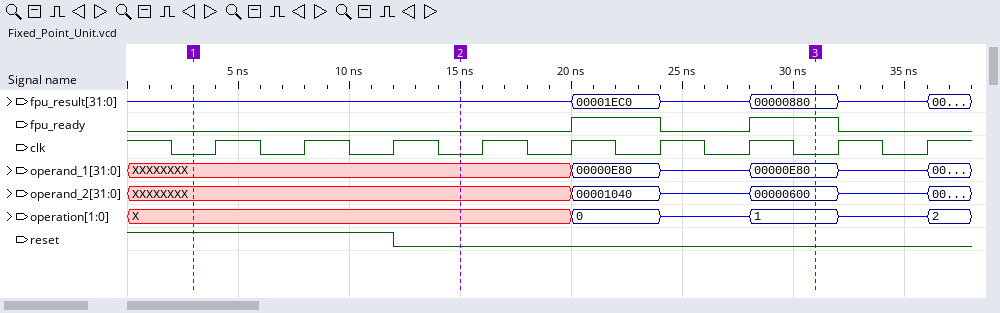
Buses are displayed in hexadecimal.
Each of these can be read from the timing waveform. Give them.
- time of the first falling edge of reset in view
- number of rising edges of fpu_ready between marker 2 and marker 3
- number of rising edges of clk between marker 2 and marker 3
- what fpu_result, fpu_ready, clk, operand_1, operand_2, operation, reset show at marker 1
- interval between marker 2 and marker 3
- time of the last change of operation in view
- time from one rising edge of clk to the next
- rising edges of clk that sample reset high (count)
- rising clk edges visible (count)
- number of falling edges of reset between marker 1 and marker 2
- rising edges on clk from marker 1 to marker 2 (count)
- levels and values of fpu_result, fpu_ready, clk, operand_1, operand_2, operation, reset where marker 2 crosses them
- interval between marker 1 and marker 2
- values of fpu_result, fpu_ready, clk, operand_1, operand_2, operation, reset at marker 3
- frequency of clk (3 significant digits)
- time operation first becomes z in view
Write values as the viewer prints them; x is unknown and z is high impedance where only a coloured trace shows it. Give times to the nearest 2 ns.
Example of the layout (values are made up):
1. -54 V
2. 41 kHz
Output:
1. 12 ns
2. 2
3. 4
4. fpu_result=z, fpu_ready=0, clk=0, operand_1=XXXXXXXX, operand_2=XXXXXXXX, operation=X, reset=1
5. 16 ns
6. 36 ns
7. 4 ns
8. 3
9. 9
10. 1
11. 3
12. fpu_result=z, fpu_ready=0, clk=0, operand_1=XXXXXXXX, operand_2=XXXXXXXX, operation=X, reset=0
13. 12 ns
14. fpu_result=00000880, fpu_ready=1, clk=0, operand_1=00000E80, operand_2=00000600, operation=1, reset=0
15. 250 MHz
16. 24 ns
